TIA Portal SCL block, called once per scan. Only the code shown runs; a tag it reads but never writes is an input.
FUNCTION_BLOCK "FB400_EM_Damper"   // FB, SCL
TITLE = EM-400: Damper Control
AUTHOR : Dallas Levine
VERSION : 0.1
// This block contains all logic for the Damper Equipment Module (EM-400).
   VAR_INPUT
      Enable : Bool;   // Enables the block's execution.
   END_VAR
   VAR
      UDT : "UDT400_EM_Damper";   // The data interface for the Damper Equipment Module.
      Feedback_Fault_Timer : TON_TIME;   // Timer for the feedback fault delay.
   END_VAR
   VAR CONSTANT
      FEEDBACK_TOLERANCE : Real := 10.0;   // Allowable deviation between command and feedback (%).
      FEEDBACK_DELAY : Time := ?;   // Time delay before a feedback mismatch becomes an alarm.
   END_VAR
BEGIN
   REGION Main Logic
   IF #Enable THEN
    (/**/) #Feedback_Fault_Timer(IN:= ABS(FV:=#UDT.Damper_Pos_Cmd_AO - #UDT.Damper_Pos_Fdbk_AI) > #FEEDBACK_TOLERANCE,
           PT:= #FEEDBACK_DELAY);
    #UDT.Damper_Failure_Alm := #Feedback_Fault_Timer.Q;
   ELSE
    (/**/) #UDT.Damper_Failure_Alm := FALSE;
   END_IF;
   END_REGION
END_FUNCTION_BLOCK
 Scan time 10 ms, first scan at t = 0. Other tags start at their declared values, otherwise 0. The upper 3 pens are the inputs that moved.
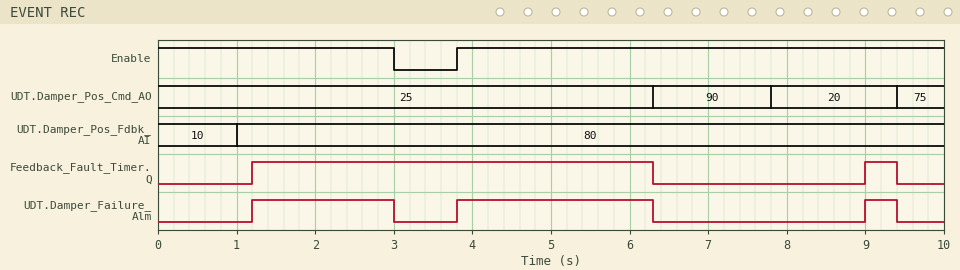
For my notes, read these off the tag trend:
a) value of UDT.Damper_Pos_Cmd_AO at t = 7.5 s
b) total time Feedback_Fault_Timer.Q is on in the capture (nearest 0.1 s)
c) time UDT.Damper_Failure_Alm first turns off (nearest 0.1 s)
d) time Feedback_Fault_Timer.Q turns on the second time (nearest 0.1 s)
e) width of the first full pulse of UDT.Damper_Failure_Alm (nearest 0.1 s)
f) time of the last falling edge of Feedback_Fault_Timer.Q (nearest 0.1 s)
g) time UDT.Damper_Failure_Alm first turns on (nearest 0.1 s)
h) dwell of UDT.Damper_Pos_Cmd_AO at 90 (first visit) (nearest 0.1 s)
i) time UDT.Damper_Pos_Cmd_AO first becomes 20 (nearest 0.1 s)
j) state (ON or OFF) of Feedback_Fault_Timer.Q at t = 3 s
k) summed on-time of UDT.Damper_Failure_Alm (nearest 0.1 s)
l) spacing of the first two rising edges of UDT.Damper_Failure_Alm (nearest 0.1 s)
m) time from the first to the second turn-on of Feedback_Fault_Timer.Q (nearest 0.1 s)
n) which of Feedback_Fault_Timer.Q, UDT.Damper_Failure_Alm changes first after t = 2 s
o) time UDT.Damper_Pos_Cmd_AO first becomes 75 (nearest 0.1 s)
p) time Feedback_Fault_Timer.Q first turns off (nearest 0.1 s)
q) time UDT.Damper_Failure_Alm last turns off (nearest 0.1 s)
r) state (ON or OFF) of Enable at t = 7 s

90
5.5 s
3.0 s
9.0 s
1.8 s
9.4 s
1.2 s
1.5 s
7.8 s
ON
4.7 s
2.6 s
7.8 s
UDT.Damper_Failure_Alm
9.4 s
6.3 s
9.4 s
ON
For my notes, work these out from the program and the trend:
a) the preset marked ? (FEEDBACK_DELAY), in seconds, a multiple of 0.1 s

1.2 s
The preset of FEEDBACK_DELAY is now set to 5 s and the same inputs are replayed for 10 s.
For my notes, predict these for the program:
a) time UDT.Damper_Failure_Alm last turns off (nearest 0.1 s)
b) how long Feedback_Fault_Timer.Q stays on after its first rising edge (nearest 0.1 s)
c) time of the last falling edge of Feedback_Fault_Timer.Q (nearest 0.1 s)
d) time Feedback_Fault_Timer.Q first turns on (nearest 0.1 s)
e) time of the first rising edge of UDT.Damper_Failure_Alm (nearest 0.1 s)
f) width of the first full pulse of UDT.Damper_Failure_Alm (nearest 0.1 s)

6.3 s
1.3 s
6.3 s
5.0 s
5.0 s
1.3 s
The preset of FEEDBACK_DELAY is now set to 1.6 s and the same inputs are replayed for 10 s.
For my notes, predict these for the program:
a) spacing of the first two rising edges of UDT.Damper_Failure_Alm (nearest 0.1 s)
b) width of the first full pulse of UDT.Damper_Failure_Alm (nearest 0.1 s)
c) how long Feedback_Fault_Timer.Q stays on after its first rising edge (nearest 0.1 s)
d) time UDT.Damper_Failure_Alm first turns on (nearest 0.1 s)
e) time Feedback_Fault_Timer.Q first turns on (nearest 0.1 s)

2.2 s
1.4 s
4.7 s
1.6 s
1.6 s
